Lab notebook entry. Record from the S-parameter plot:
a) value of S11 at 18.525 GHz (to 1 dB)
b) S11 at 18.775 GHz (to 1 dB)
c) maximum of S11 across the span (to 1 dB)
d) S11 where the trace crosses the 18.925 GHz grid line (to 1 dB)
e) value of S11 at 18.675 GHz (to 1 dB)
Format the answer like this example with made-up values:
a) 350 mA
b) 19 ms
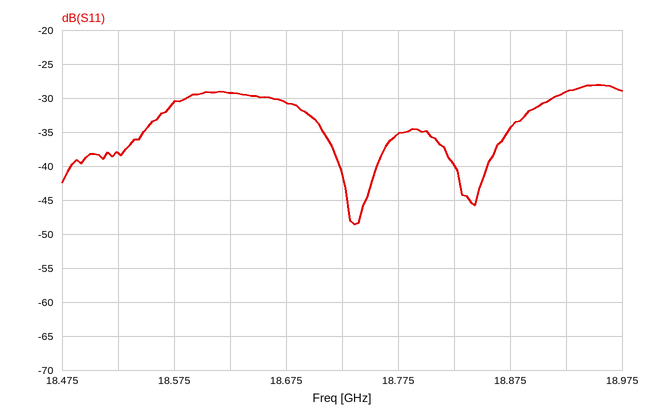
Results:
a) -38 dB
b) -35 dB
c) -28 dB
d) -29 dB
e) -31 dB
